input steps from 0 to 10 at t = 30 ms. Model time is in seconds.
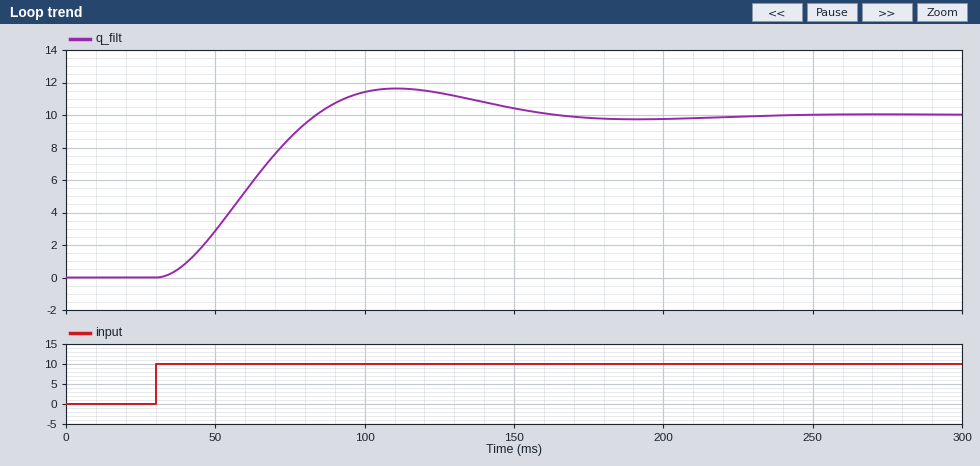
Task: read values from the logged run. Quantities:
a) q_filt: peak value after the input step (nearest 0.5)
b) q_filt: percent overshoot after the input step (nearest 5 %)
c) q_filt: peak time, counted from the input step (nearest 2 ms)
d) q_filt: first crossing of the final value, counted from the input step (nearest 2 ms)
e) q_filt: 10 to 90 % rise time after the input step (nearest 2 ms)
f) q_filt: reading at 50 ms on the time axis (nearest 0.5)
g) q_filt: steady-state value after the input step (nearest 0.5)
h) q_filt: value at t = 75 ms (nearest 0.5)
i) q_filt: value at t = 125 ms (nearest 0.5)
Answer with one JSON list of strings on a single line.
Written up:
["11.5", "15 %", "80 ms", "54 ms", "36 ms", "3.0", "10.0", "8.5", "11.5"]
